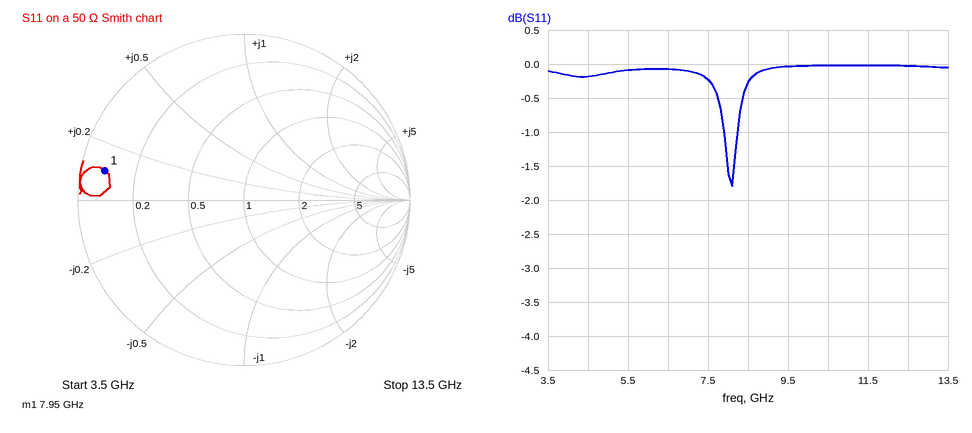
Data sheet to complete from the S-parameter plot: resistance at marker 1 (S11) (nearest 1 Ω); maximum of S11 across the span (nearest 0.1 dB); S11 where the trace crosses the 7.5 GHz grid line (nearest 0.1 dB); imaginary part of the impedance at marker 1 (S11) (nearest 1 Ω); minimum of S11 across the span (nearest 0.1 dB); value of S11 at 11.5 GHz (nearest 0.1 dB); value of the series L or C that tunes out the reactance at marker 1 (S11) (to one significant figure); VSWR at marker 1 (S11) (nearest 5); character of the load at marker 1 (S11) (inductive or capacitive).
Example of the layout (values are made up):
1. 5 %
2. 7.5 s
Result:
1. 4 Ω
2. 0.0 dB
3. -0.2 dB
4. +5 Ω
5. -1.8 dB
6. 0.0 dB
7. 4 pF
8. 15
9. inductive
